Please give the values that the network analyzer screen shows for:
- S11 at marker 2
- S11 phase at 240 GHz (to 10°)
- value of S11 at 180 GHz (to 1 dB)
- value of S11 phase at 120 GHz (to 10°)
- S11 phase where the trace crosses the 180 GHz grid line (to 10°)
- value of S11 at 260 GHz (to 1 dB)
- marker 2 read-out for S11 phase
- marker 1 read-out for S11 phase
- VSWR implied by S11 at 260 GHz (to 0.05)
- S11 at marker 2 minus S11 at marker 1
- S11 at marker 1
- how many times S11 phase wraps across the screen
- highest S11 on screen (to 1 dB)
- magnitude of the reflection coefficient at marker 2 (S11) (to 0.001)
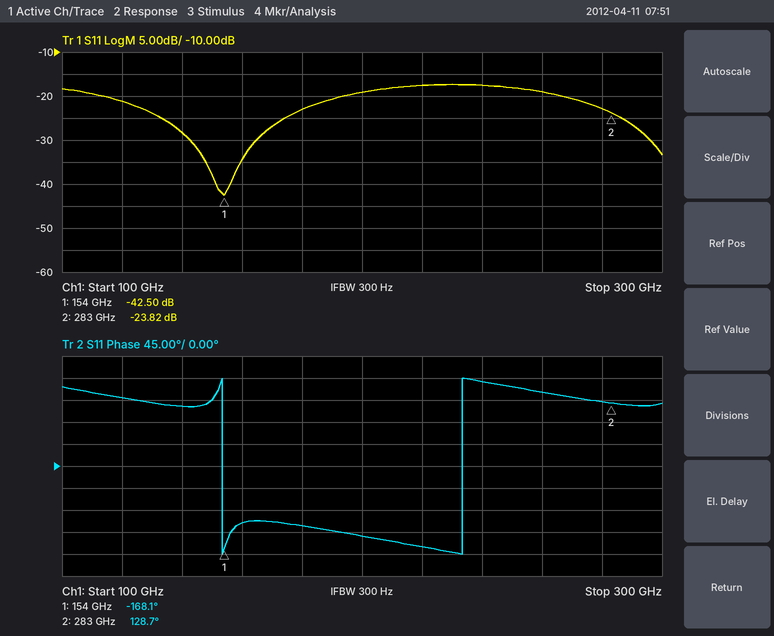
-23.82 dB
170°
-23 dB
140°
-120°
-19 dB
128.7°
-168.1°
1.25
18.68 dB
-42.50 dB
2
-17 dB
0.064
